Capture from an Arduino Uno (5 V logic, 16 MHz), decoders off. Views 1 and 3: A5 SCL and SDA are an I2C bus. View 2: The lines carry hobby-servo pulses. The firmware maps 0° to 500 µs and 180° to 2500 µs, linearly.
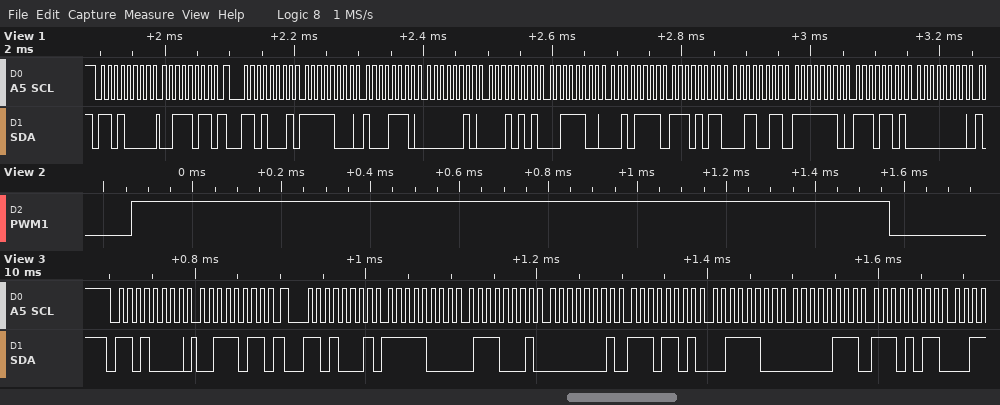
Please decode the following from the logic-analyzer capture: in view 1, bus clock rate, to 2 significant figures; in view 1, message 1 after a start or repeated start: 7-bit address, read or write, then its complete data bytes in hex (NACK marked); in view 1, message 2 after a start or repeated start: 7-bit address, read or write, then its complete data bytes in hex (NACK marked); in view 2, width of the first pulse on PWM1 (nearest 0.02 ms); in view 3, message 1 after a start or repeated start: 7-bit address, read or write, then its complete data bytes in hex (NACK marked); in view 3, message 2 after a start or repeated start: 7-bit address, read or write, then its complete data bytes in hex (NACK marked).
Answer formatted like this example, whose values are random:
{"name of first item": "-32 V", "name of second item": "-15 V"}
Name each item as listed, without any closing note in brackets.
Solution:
{"in view 1, bus clock rate, to 2 significant figures": "100 kHz", "in view 1, message 1 after a start or repeated start: 7-bit address, read or write, then its complete data bytes in hex": "0x68 write: 3B", "in view 1, message 2 after a start or repeated start: 7-bit address, read or write, then its complete data bytes in hex": "0x68 read: F8 8E 02 15 3C 2F EB 33 FE ED 00", "in view 2, width of the first pulse on PWM1": "1.70 ms", "in view 3, message 1 after a start or repeated start: 7-bit address, read or write, then its complete data bytes in hex": "0x68 write: 3B", "in view 3, message 2 after a start or repeated start: 7-bit address, read or write, then its complete data bytes in hex": "0x68 read: F8 71 01 ED 3C 07 EB"}
